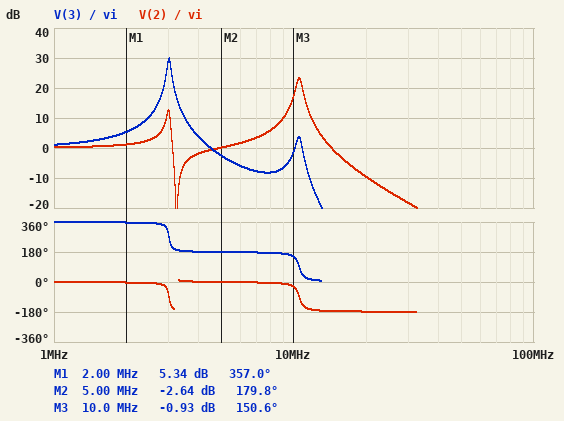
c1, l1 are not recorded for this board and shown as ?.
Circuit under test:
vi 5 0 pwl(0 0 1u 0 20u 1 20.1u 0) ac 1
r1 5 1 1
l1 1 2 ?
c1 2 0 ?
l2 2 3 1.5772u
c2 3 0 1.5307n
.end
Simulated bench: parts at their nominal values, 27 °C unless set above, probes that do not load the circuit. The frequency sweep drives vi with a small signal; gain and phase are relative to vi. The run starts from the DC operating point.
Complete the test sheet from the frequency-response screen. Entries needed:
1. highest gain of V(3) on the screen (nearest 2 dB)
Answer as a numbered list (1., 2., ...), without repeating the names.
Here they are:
1. 30 dB
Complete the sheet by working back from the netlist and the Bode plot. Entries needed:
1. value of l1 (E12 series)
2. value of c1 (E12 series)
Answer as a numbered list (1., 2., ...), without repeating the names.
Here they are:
1. 220 nH
2. 1.2 nF
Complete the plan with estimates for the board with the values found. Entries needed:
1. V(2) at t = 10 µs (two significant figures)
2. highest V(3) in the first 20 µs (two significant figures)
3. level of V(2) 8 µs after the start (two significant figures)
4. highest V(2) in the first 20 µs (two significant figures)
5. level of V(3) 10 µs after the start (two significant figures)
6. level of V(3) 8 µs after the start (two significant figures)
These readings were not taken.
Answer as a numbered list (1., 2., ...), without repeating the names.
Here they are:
1. 470 mV
2. 1.0 V
3. 370 mV
4. 1.0 V
5. 470 mV
6. 370 mV
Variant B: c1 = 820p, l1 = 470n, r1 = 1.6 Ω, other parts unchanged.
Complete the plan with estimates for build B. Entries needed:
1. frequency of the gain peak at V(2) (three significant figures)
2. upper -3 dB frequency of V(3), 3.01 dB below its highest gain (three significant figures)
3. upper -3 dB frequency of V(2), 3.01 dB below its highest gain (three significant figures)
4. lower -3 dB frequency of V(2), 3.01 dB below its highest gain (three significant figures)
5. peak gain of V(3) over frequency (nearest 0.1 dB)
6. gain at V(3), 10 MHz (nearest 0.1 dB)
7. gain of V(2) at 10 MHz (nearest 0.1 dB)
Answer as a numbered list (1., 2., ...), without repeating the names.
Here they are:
1. 9.37 MHz
2. 2.87 MHz
3. 9.57 MHz
4. 9.17 MHz
5. 26.2 dB
6. -4.6 dB
7. 14.0 dB
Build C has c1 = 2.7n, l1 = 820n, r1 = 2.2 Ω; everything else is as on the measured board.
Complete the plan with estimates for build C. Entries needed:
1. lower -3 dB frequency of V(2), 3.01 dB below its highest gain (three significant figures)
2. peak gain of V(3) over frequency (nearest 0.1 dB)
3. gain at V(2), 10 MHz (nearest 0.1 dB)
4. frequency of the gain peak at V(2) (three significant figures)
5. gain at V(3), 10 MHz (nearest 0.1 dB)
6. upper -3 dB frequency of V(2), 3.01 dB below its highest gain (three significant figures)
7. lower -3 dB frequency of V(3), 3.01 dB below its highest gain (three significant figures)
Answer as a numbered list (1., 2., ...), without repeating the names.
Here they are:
1. 4.67 MHz
2. 20.8 dB
3. -17.1 dB
4. 4.74 MHz
5. -35.7 dB
6. 4.82 MHz
7. 2.17 MHz
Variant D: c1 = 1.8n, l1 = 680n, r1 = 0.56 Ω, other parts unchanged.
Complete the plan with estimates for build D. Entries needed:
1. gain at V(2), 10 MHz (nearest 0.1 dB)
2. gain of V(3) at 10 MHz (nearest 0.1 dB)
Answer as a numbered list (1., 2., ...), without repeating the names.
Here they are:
1. -10.5 dB
2. -29.1 dB
